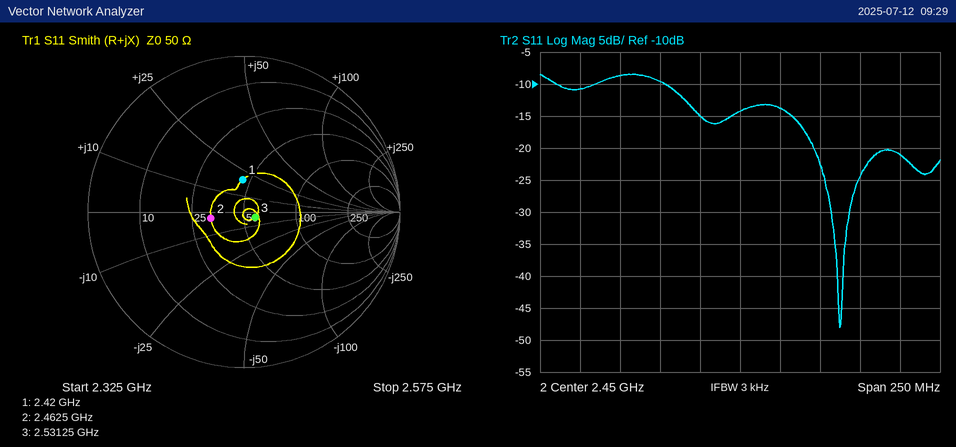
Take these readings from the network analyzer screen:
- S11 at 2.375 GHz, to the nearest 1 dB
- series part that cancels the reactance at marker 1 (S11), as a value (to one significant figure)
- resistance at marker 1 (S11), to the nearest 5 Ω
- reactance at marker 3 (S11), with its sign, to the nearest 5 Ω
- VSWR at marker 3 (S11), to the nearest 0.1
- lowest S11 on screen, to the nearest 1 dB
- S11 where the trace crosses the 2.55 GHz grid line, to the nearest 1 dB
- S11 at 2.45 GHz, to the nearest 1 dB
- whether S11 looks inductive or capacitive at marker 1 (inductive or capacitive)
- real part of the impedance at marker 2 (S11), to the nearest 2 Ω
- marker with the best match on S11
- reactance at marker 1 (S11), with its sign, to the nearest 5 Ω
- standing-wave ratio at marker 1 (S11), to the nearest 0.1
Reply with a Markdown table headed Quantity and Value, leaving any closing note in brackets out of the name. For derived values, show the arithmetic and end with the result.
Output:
| Quantity | Value |
|---|---|
| S11 at 2.375 GHz, to the nearest 1 dB | -9 dB |
| series part that cancels the reactance at marker 1 (S11), as a value | C = 1/(2π × 2.42 GHz × 20 Ω) ≈ 3 pF |
| resistance at marker 1 (S11), to the nearest 5 Ω | 45 Ω |
| reactance at marker 3 (S11), with its sign, to the nearest 5 Ω | -5 Ω |
| VSWR at marker 3 (S11), to the nearest 0.1 | 1.2 |
| lowest S11 on screen, to the nearest 1 dB | -48 dB |
| S11 where the trace crosses the 2.55 GHz grid line, to the nearest 1 dB | -21 dB |
| S11 at 2.45 GHz, to the nearest 1 dB | -14 dB |
| whether S11 looks inductive or capacitive at marker 1 | inductive |
| real part of the impedance at marker 2 (S11), to the nearest 2 Ω | 32 Ω |
| marker with the best match on S11 | marker 3 |
| reactance at marker 1 (S11), with its sign, to the nearest 5 Ω | +20 Ω |
| standing-wave ratio at marker 1 (S11), to the nearest 0.1 | 1.5 |
